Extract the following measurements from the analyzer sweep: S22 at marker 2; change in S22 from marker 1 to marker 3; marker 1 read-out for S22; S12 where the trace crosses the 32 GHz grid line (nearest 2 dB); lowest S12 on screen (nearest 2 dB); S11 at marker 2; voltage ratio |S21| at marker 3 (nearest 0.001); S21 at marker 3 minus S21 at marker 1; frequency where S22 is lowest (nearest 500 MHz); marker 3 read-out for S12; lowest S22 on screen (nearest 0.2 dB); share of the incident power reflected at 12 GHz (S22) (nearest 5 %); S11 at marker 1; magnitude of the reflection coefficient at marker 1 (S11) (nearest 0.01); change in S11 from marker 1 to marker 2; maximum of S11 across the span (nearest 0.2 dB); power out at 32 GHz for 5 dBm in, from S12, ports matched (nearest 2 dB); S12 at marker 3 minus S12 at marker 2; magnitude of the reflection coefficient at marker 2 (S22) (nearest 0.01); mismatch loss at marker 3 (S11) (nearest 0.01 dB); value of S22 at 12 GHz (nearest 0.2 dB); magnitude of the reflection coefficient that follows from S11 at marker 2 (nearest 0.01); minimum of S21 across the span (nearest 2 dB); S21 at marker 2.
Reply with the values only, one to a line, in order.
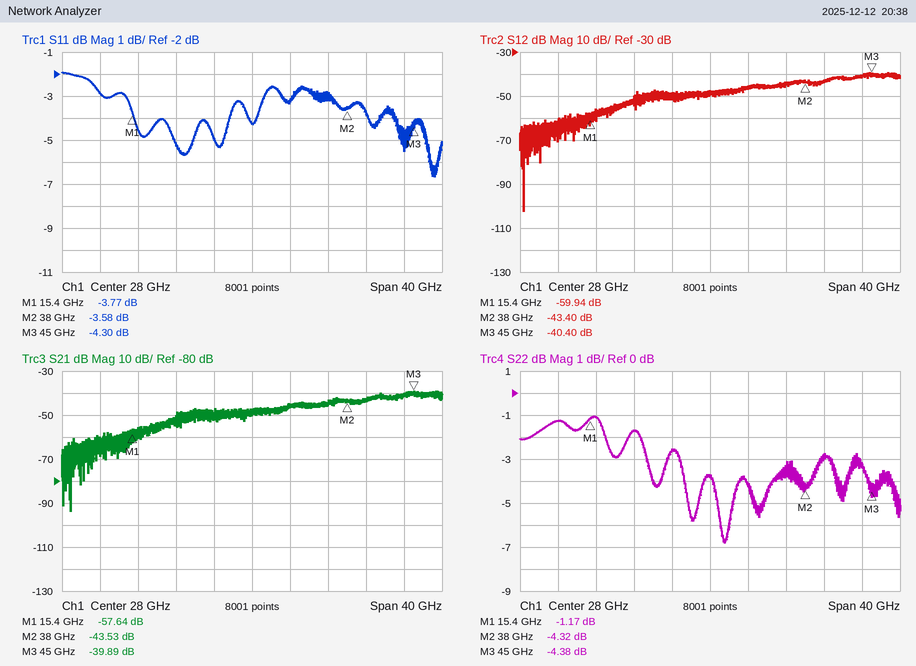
-4.32 dB
-3.21 dB
-1.17 dB
-46 dB
-102 dB
-3.58 dB
0.010
17.75 dB
29.5 GHz
-40.40 dB
-6.8 dB
75 %
-3.77 dB
0.65
0.19 dB
-2.0 dB
-42 dBm
3.00 dB
0.61
2.02 dB
-1.2 dB
0.66
-94 dB
-43.53 dB
